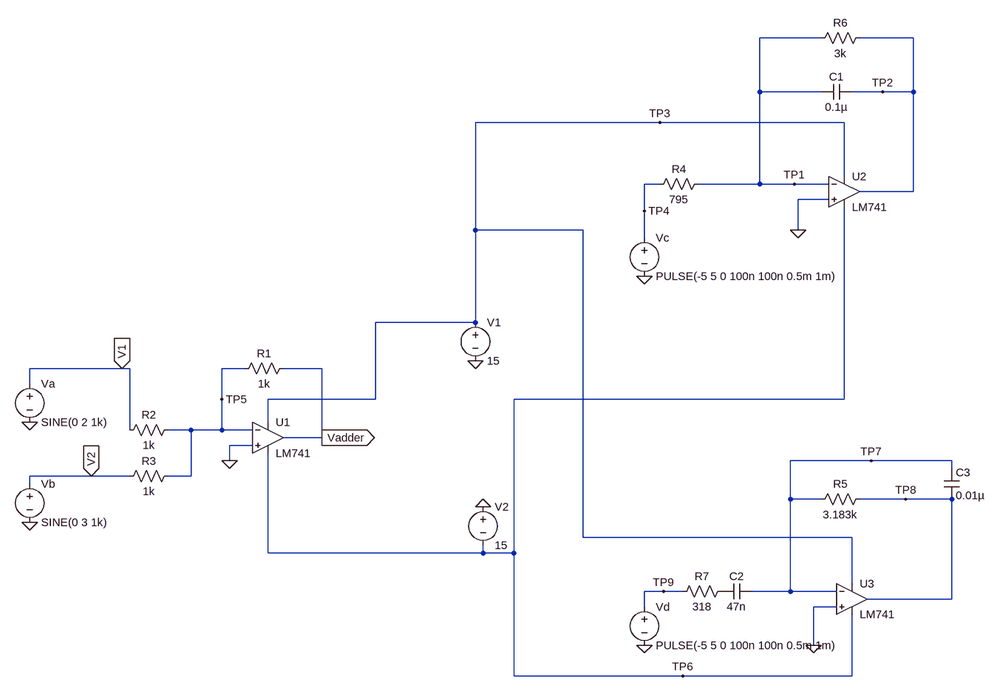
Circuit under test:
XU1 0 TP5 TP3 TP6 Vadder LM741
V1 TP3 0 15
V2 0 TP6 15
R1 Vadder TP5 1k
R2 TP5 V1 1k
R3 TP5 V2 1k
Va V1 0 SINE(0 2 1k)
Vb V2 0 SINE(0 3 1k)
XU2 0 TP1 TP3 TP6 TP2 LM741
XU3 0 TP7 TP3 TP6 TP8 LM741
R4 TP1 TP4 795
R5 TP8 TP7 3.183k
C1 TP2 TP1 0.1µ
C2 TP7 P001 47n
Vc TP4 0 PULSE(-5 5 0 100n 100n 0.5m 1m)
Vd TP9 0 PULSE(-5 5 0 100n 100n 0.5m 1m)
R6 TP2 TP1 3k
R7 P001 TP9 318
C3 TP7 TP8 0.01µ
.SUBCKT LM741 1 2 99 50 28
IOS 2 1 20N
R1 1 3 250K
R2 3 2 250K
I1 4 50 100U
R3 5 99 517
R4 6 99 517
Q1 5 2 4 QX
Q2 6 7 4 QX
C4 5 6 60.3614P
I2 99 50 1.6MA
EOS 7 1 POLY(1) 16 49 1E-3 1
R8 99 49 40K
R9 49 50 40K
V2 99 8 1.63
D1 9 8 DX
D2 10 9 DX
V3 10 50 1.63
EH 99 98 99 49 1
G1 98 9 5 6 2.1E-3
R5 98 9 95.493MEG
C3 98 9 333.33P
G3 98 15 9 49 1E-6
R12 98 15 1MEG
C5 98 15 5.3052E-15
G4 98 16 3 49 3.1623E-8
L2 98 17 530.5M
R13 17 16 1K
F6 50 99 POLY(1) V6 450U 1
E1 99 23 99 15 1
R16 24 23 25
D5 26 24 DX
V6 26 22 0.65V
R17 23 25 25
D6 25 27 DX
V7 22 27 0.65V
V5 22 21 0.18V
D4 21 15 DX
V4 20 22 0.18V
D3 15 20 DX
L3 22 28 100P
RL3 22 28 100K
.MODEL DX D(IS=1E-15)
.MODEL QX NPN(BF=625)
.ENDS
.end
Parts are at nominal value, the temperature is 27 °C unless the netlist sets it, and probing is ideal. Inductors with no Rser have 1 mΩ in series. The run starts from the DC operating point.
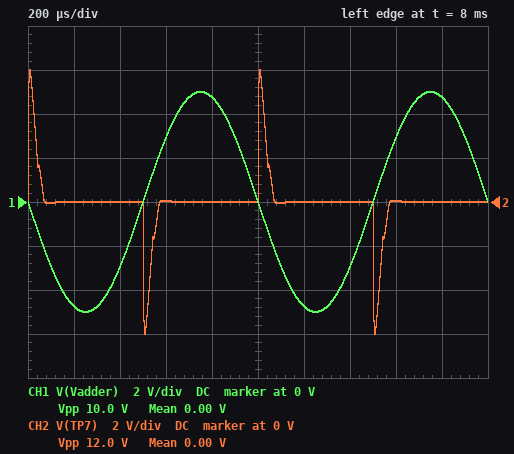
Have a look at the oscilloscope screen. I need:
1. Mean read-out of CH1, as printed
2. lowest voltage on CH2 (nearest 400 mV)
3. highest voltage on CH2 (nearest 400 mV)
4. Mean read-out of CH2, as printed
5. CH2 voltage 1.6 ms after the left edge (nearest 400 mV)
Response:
0.00 V
-6.0 V
6.0 V
0.00 V
0 V
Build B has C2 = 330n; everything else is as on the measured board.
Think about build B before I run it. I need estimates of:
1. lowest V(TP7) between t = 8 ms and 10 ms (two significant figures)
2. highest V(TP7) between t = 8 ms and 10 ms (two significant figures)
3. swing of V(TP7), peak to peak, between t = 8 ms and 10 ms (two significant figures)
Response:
-7.7 V
7.7 V
15 V
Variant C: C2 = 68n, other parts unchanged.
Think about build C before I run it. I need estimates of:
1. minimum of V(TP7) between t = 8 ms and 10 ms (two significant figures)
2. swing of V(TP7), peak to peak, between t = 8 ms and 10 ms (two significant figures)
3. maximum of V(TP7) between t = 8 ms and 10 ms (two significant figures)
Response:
-6.4 V
13 V
6.4 V
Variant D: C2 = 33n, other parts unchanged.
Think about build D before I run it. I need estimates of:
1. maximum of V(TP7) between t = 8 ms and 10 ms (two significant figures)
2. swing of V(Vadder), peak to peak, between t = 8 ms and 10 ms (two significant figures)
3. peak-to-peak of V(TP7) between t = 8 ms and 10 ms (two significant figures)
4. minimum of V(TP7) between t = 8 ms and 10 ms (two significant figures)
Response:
5.5 V
10 V
11 V
-5.5 V
